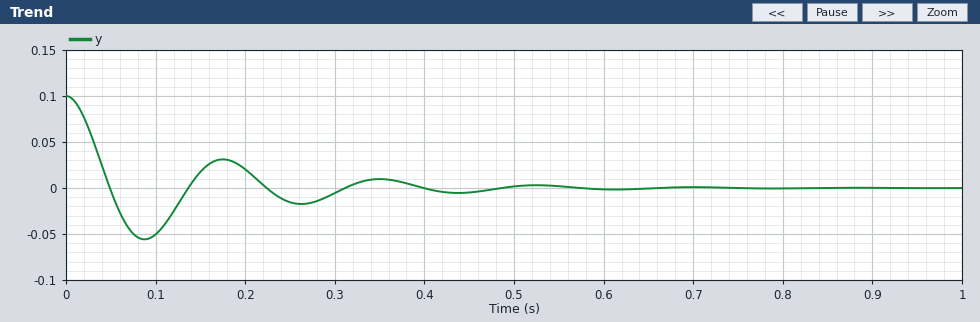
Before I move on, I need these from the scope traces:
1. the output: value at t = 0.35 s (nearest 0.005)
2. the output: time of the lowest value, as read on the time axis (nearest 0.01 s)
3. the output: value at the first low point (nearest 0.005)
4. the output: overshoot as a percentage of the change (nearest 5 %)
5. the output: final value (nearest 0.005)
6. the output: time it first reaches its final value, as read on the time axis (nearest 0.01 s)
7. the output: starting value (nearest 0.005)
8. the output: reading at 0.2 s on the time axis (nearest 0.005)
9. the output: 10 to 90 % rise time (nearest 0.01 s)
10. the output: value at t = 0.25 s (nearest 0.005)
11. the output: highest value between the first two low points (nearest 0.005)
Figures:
0.010
0.09 s
-0.055
55 %
0.000
0.05 s
0.100
0.020
0.03 s
-0.015
0.030
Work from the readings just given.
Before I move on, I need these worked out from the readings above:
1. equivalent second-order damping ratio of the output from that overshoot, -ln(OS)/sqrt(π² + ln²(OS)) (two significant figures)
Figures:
0.19
